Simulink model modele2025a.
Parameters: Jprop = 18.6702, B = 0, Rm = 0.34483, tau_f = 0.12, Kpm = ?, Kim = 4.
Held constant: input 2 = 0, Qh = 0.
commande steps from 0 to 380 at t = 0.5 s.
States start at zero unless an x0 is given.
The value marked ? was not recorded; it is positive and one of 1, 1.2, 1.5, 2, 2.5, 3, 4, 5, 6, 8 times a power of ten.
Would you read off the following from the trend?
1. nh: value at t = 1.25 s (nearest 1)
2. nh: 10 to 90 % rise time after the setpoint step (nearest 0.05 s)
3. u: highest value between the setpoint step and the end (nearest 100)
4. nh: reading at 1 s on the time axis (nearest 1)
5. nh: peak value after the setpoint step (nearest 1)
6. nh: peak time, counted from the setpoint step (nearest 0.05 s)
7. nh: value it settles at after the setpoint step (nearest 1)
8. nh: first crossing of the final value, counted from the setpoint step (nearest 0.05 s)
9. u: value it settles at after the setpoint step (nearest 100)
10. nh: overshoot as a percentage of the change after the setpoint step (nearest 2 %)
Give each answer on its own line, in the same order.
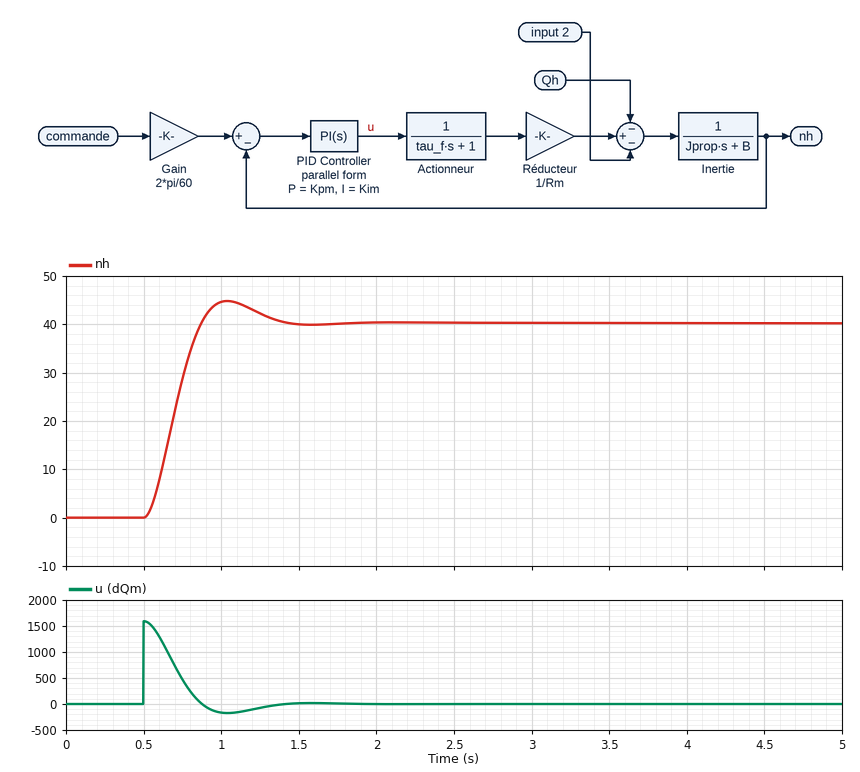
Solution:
42
0.25 s
1600
45
45
0.55 s
40
0.35 s
0
12 %
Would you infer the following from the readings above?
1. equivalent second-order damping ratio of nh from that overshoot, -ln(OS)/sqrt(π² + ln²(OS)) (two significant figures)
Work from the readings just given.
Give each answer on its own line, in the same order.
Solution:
0.56
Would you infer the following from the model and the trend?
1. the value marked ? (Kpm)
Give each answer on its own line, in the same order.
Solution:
40
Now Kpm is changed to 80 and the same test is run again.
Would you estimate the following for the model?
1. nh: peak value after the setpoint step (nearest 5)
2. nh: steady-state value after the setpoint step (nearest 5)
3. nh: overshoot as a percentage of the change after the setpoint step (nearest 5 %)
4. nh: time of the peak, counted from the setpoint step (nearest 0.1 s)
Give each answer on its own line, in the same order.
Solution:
50
40
25 %
0.3 s
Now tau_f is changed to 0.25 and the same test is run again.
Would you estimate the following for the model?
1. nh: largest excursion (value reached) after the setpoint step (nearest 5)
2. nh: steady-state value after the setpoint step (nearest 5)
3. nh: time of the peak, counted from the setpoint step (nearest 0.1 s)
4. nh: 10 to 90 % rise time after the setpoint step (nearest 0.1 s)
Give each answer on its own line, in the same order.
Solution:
50
40
0.7 s
0.3 s
